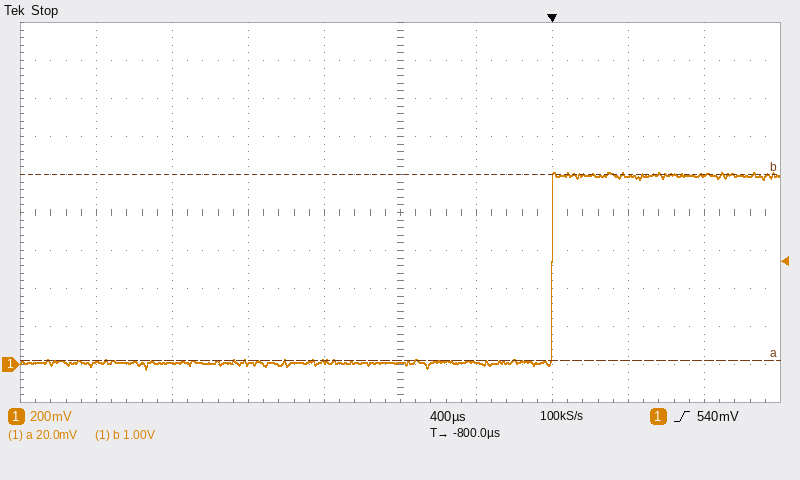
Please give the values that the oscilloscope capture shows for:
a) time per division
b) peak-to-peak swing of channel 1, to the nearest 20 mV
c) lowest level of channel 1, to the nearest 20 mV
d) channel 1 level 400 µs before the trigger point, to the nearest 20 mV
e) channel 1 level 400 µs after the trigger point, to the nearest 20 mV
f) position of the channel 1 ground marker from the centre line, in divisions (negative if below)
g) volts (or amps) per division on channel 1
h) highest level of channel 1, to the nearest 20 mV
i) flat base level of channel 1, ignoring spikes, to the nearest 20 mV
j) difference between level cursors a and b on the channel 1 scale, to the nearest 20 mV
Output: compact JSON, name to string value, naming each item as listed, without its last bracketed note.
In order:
{"time per division": "400 µs", "peak-to-peak swing of channel 1, to the nearest 20 mV": "1.04 V", "lowest level of channel 1, to the nearest 20 mV": "-20 mV", "channel 1 level 400 µs before the trigger point, to the nearest 20 mV": "20 mV", "channel 1 level 400 µs after the trigger point, to the nearest 20 mV": "1.00 V", "position of the channel 1 ground marker from the centre line, in divisions": "-4.0 div", "volts (or amps) per division on channel 1": "200 mV", "highest level of channel 1, to the nearest 20 mV": "1.02 V", "flat base level of channel 1, ignoring spikes, to the nearest 20 mV": "20 mV", "difference between level cursors a and b on the channel 1 scale, to the nearest 20 mV": "980 mV"}
